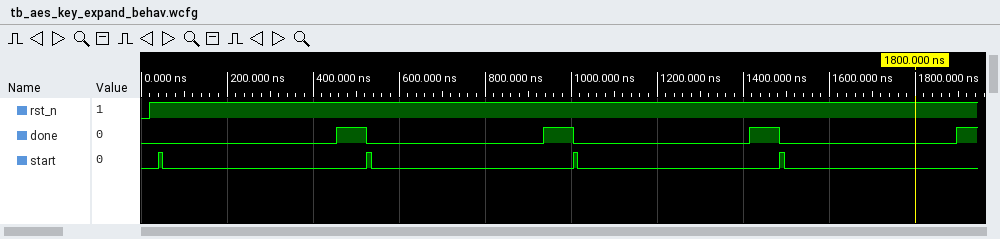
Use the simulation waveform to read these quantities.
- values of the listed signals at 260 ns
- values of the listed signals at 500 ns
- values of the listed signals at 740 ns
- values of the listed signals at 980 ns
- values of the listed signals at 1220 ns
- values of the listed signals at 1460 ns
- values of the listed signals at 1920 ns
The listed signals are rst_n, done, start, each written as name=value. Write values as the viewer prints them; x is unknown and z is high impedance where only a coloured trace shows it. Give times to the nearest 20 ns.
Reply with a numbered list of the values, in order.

1. rst_n=1, done=0, start=0
2. rst_n=1, done=1, start=0
3. rst_n=1, done=0, start=0
4. rst_n=1, done=1, start=0
5. rst_n=1, done=0, start=0
6. rst_n=1, done=1, start=0
7. rst_n=1, done=1, start=0
